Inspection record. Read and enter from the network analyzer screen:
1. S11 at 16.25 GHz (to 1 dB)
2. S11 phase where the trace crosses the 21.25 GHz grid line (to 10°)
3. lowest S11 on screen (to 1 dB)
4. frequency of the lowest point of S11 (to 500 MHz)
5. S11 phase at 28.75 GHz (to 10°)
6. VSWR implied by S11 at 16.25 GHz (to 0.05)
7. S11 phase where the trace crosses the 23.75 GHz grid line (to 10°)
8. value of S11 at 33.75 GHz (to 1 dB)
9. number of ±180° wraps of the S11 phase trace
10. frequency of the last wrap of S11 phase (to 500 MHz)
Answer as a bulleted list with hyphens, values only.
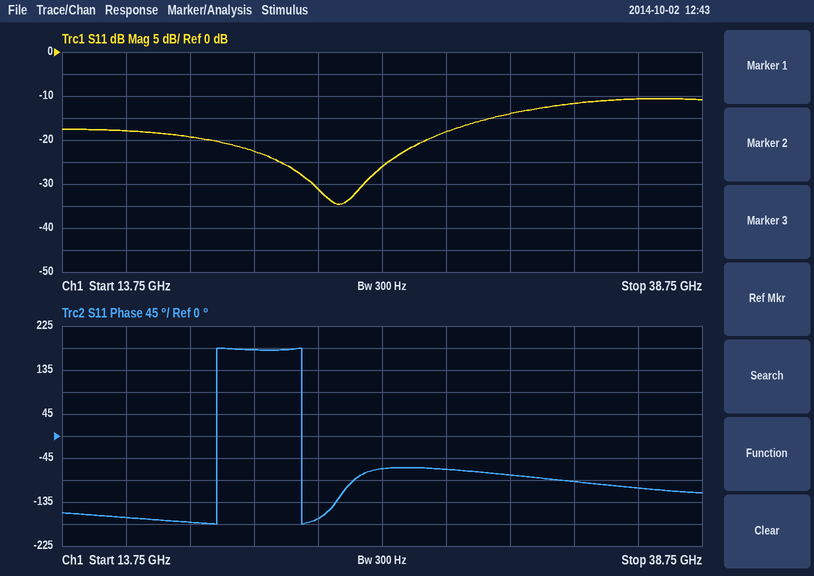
- -18 dB
- 180°
- -35 dB
- 24.5 GHz
- -70°
- 1.30
- -170°
- -12 dB
- 2
- 23.0 GHz
